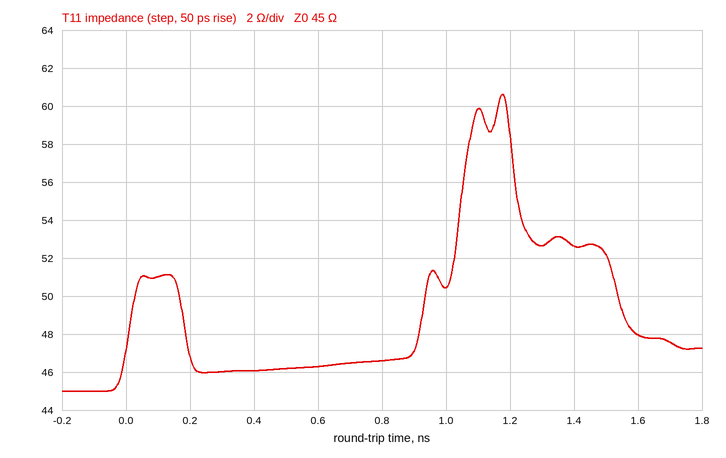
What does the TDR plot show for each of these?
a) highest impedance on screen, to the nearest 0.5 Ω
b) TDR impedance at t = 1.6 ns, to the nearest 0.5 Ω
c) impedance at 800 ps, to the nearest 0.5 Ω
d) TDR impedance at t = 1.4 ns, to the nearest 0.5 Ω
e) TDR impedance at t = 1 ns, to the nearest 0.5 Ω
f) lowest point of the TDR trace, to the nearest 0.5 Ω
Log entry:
60.5 Ω
48.0 Ω
46.5 Ω
52.5 Ω
50.5 Ω
45.0 Ω
